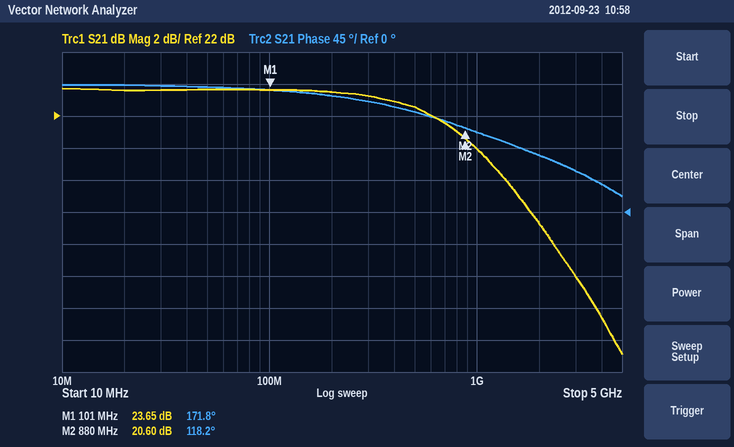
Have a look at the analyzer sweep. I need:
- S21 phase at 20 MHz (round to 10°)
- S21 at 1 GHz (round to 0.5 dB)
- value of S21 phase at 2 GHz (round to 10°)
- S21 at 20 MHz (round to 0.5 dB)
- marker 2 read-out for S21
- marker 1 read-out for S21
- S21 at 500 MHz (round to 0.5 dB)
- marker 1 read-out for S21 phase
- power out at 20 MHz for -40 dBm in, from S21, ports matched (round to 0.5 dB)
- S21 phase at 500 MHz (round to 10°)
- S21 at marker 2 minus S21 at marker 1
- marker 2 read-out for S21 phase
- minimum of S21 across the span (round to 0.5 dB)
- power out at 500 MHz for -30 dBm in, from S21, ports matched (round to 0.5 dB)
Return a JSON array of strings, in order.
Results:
["180°", "20.0 dB", "80°", "23.5 dB", "20.60 dB", "23.65 dB", "22.5 dB", "171.8°", "-16.5 dBm", "140°", "-3.05 dB", "118.2°", "7.0 dB", "-7.5 dBm"]
